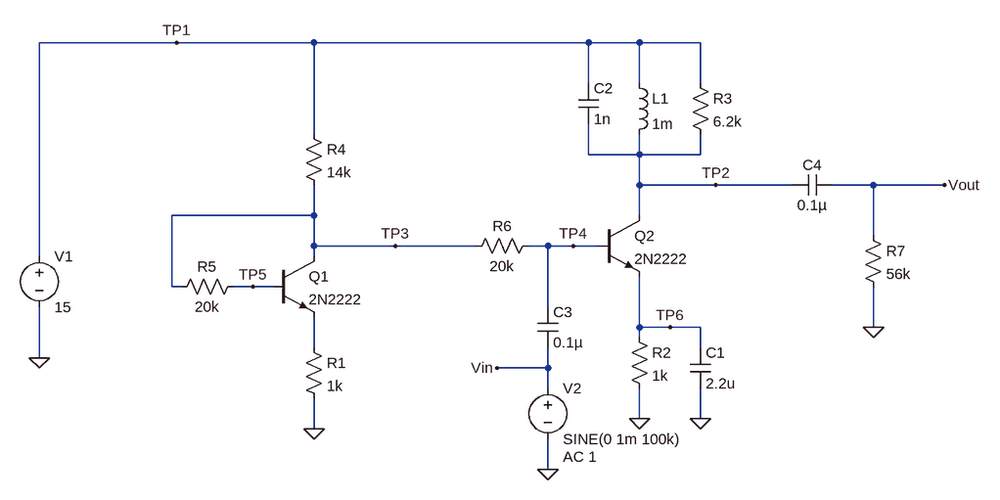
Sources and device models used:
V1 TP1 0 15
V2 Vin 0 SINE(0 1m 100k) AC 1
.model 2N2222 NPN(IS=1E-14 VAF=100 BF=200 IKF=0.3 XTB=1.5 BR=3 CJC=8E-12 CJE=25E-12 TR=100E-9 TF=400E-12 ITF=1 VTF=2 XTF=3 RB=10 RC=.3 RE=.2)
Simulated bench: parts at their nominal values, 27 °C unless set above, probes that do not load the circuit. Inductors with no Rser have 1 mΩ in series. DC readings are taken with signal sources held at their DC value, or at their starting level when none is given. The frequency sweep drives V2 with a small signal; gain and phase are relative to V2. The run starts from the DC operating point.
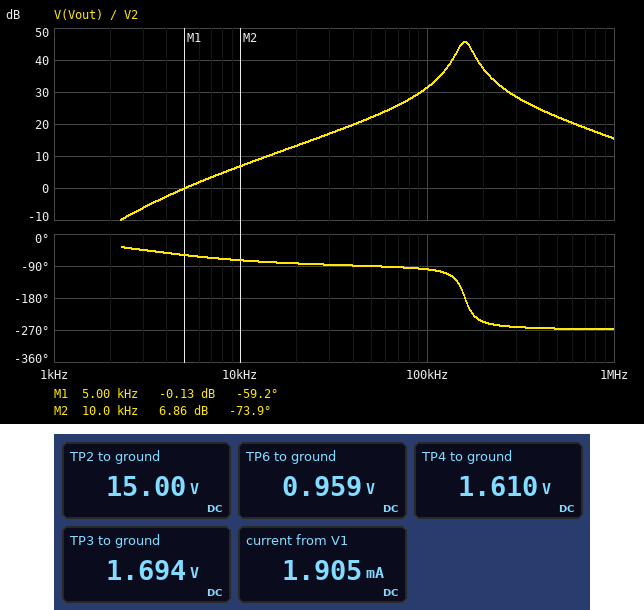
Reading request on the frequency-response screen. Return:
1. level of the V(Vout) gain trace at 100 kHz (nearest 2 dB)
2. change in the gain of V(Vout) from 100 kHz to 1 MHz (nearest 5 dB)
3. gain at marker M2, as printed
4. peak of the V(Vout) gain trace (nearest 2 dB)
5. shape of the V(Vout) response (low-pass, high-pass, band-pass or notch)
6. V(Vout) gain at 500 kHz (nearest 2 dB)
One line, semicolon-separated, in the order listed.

32 dB; -15 dB; 6.86 dB; 46 dB; band-pass; 22 dB
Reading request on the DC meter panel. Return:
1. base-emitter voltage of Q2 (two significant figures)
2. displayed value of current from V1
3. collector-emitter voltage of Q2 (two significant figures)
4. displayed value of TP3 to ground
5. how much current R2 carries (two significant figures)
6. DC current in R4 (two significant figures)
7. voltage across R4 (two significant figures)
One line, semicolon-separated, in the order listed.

650 mV; 1.905 mA; 14 V; 1.694 V; 960 µA; 950 µA; 13 V
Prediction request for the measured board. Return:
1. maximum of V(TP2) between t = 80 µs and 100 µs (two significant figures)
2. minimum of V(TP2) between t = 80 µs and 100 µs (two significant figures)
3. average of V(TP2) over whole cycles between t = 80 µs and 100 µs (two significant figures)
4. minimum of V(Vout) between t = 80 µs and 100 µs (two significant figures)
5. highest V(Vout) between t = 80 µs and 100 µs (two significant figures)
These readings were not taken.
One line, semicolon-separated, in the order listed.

15 V; 15 V; 15 V; -37 mV; 38 mV
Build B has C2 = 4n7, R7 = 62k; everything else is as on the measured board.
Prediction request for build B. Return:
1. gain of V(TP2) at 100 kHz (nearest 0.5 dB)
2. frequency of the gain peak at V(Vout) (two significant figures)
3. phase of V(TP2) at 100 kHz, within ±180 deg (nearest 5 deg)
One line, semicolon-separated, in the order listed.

28.5 dB; 73 kHz; 100 deg
